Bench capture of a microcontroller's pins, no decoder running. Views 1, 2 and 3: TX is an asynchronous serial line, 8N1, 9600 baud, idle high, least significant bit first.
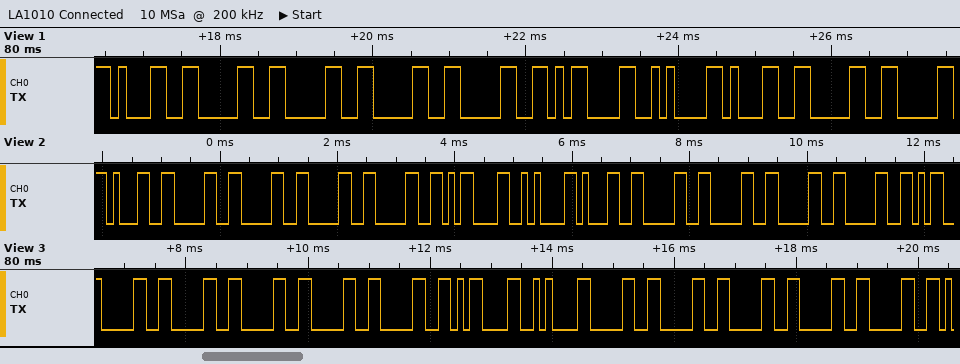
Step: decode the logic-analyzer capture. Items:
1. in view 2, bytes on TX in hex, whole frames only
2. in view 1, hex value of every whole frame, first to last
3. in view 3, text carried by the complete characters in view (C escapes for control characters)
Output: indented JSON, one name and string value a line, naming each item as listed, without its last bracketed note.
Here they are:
{
  "in view 2, bytes on TX in hex, whole frames only": "31 30 30 30 30 0D 0A 31 30 30 30 30",
  "in view 1, hex value of every whole frame, first to last": "31 30 30 30 30 0D 0A 31 30",
  "in view 3, text carried by the complete characters in view": "\"00000\\r\\n00000\""
}
